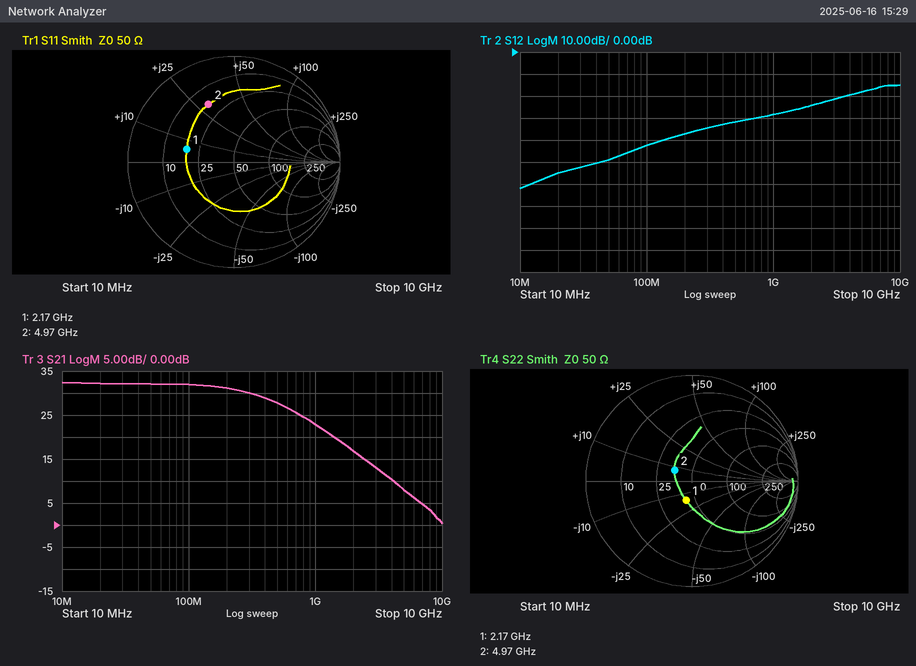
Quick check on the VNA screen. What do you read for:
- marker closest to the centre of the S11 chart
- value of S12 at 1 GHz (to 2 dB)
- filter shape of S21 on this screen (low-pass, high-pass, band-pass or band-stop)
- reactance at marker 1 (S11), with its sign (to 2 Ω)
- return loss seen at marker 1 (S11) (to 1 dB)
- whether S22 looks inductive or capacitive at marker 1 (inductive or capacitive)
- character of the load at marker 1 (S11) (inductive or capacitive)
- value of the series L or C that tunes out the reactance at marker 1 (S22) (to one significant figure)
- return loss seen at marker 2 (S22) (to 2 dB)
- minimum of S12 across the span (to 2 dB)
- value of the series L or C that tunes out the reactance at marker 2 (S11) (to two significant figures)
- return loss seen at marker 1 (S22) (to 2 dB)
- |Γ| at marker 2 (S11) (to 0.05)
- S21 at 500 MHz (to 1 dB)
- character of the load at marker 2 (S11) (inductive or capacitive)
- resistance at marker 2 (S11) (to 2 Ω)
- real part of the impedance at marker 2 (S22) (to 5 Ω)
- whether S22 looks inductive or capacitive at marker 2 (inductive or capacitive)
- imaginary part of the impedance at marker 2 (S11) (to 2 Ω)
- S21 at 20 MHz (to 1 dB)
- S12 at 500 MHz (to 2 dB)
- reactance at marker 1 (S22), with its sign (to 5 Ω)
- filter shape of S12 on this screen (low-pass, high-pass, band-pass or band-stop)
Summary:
marker 1
-28 dB
low-pass
+6 Ω
7 dB
capacitive
inductive
1 nH
14 dB
-62 dB
1.1 pF
14 dB
0.60
28 dB
inductive
18 Ω
35 Ω
inductive
+30 Ω
32 dB
-32 dB
-15 Ω
high-pass
